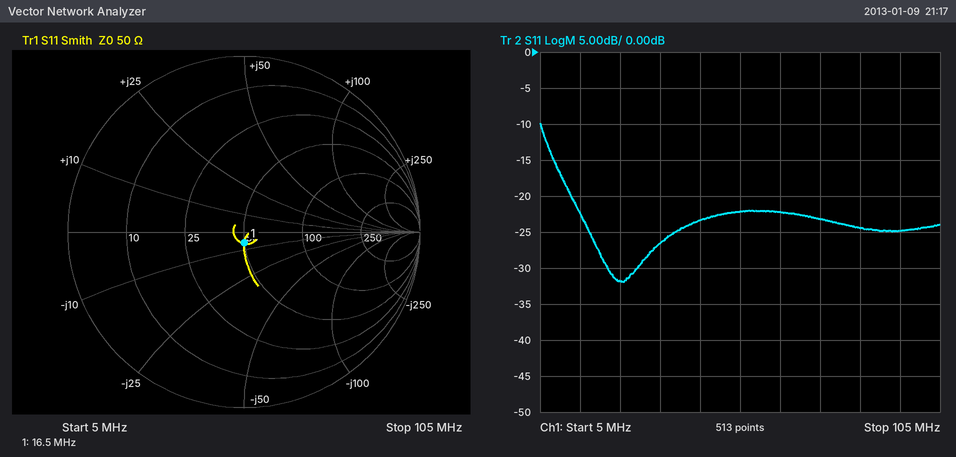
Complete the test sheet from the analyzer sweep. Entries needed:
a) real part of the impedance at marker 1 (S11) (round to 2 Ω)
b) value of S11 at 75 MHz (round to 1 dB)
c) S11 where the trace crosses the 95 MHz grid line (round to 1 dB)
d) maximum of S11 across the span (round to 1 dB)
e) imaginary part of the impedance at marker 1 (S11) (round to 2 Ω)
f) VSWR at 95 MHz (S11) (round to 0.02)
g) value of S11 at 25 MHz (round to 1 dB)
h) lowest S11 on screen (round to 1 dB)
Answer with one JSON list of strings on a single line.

["50 Ω", "-23 dB", "-25 dB", "-10 dB", "-6 Ω", "1.12", "-32 dB", "-32 dB"]
